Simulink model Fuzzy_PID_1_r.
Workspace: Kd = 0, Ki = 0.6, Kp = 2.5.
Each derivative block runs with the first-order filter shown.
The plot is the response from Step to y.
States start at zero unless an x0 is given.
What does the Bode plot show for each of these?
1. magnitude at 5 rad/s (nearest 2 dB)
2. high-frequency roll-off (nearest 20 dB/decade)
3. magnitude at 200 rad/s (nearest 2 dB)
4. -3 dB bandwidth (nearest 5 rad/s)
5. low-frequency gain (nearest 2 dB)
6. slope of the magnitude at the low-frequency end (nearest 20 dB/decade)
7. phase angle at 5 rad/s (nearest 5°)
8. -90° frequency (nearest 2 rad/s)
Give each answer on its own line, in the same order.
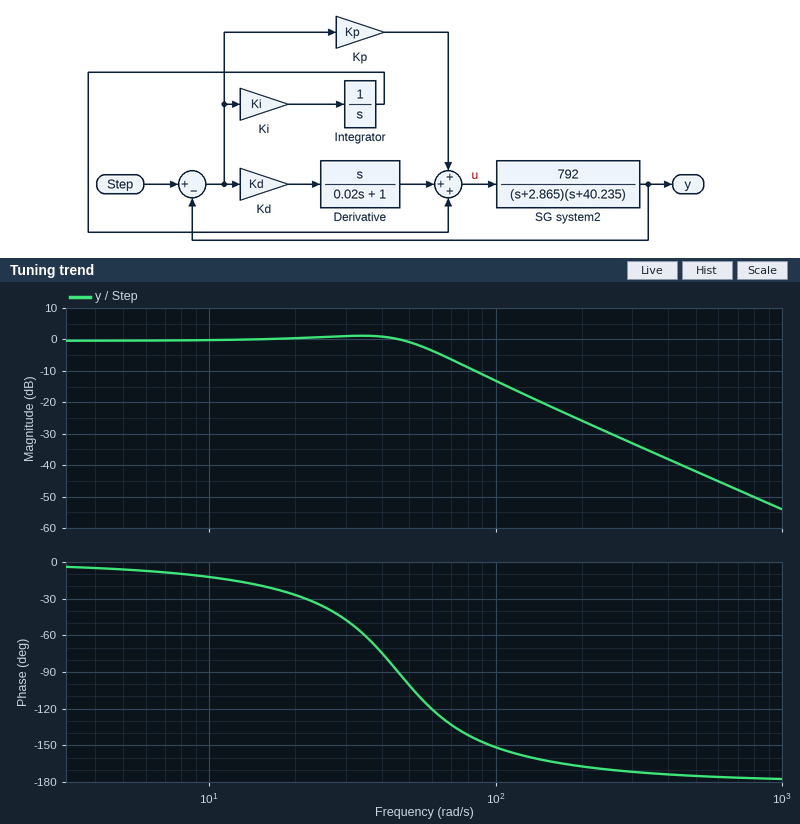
0 dB
-40 dB/decade
-26 dB
60 rad/s
0 dB
0 dB/decade
-5°
46 rad/s
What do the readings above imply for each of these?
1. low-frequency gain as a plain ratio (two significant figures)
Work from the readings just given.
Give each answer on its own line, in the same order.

1.0
